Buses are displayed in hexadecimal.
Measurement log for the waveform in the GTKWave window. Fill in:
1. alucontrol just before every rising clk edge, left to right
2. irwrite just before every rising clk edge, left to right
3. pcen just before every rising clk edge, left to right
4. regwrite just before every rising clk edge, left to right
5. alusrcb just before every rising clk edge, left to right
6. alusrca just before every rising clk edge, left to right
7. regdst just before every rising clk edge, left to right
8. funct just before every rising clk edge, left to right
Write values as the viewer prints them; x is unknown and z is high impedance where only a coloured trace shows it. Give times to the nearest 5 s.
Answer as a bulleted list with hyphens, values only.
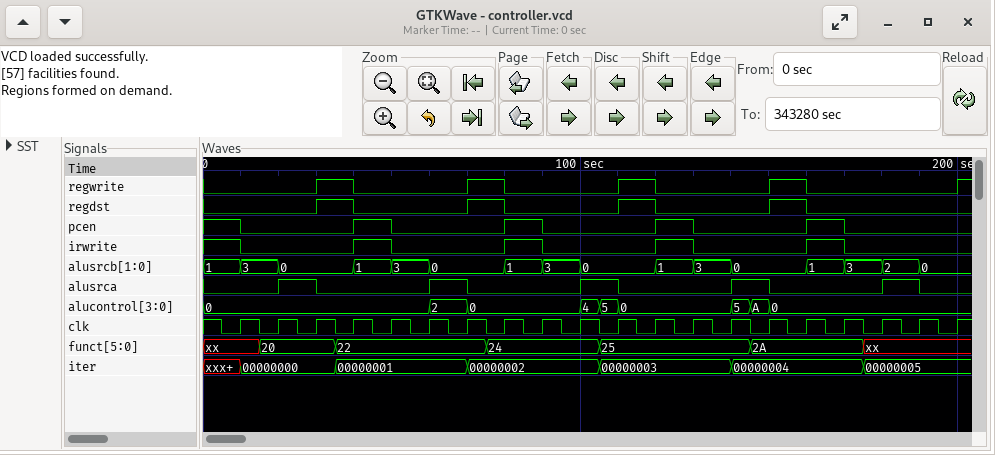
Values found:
- 0, 0, 0, 0, 0, 0, 2, 0, 0, 0, 5, 0, 0, 0, A, 0, 0, 0, 0, 0
- 1 0 0 0 1 0 0 0 1 0 0 0 1 0 0 0 1 0 0 0
- 1 0 0 0 1 0 0 0 1 0 0 0 1 0 0 0 1 0 0 0
- 0 0 0 1 0 0 0 1 0 0 0 1 0 0 0 1 0 0 0 0
- 1, 3, 0, 0, 1, 3, 0, 0, 1, 3, 0, 0, 1, 3, 0, 0, 1, 3, 2, 0
- 0 0 1 0 0 0 1 0 0 0 1 0 0 0 1 0 0 0 1 0
- 0 0 0 1 0 0 0 1 0 0 0 1 0 0 0 1 0 0 0 0
- xx, 20, 20, 22, 22, 22, 22, 24, 24, 24, 25, 25, 25, 25, 2A, 2A, 2A, xx, xx, xx
